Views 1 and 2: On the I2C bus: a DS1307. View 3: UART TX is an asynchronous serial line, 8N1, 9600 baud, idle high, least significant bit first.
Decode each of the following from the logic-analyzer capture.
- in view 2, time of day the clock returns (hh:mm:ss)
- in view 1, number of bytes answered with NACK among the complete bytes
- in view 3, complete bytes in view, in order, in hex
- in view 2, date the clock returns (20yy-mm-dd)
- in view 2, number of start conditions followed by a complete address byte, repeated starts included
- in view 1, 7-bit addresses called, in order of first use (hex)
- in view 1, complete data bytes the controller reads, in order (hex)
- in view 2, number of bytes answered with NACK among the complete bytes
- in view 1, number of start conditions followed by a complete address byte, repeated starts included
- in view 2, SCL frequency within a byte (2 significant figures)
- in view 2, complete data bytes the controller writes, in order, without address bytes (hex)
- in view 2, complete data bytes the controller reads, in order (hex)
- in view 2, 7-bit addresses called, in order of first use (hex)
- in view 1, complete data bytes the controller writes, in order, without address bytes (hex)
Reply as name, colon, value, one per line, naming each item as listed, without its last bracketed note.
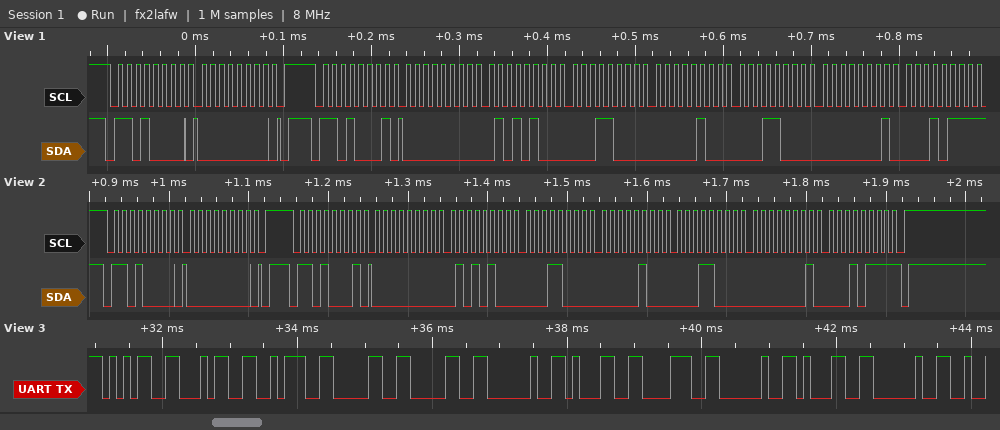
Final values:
in view 2, time of day the clock returns: 18:54:00
in view 1, number of bytes answered with NACK among the complete bytes: 1
in view 3, complete bytes in view, in order, in hex: 35 34 3A 30 30 20 31 38 20 31 20
in view 2, date the clock returns: 2017-01-18
in view 2, number of start conditions followed by a complete address byte, repeated starts included: 2
in view 1, 7-bit addresses called, in order of first use: 0x68
in view 1, complete data bytes the controller reads, in order: 00 54 18 04 18 01 17
in view 2, number of bytes answered with NACK among the complete bytes: 1
in view 1, number of start conditions followed by a complete address byte, repeated starts included: 2
in view 2, SCL frequency within a byte: 100 kHz
in view 2, complete data bytes the controller writes, in order, without address bytes: 00
in view 2, complete data bytes the controller reads, in order: 00 54 18 04 18 01 17
in view 2, 7-bit addresses called, in order of first use: 0x68
in view 1, complete data bytes the controller writes, in order, without address bytes: 00
